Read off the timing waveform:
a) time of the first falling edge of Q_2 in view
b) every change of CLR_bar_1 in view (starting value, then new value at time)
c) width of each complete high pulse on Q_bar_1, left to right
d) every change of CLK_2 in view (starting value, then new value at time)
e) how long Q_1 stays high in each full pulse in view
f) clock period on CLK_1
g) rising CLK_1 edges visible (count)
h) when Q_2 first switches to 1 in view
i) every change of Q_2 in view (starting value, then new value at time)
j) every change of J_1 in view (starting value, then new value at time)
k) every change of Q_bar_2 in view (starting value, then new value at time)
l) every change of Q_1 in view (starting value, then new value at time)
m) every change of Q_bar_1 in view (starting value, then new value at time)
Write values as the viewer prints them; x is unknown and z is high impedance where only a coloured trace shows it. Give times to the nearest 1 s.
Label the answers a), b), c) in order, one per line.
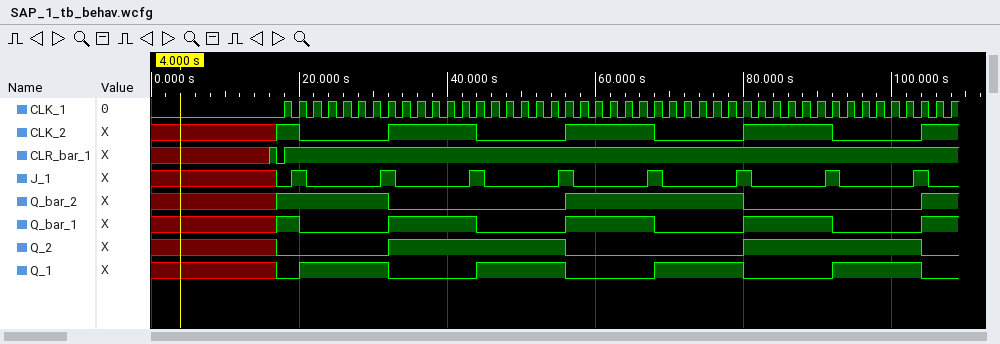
a) 56 s
b) x, 1 at 16 s, 0 at 17 s, 1 at 18 s
c) 12 s, 12 s, 12 s
d) x, 1 at 17 s, 0 at 20 s, 1 at 32 s, 0 at 44 s, 1 at 56 s, 0 at 68 s, 1 at 80 s, 0 at 92 s, 1 at 104 s
e) 12 s, 12 s, 12 s, 12 s
f) 2 s
g) 46
h) 32 s
i) x, 0 at 17 s, 1 at 32 s, 0 at 56 s, 1 at 80 s, 0 at 104 s
j) x, 0 at 17 s, 1 at 19 s, 0 at 21 s, 1 at 31 s, 0 at 33 s, 1 at 43 s, 0 at 45 s, 1 at 55 s, 0 at 57 s, 1 at 67 s, 0 at 69 s, 1 at 79 s, 0 at 81 s, 1 at 91 s, 0 at 93 s, 1 at 103 s, 0 at 105 s
k) x, 1 at 17 s, 0 at 32 s, 1 at 56 s, 0 at 80 s, 1 at 104 s
l) x, 0 at 17 s, 1 at 20 s, 0 at 32 s, 1 at 44 s, 0 at 56 s, 1 at 68 s, 0 at 80 s, 1 at 92 s, 0 at 104 s
m) x, 1 at 17 s, 0 at 20 s, 1 at 32 s, 0 at 44 s, 1 at 56 s, 0 at 68 s, 1 at 80 s, 0 at 92 s, 1 at 104 s
